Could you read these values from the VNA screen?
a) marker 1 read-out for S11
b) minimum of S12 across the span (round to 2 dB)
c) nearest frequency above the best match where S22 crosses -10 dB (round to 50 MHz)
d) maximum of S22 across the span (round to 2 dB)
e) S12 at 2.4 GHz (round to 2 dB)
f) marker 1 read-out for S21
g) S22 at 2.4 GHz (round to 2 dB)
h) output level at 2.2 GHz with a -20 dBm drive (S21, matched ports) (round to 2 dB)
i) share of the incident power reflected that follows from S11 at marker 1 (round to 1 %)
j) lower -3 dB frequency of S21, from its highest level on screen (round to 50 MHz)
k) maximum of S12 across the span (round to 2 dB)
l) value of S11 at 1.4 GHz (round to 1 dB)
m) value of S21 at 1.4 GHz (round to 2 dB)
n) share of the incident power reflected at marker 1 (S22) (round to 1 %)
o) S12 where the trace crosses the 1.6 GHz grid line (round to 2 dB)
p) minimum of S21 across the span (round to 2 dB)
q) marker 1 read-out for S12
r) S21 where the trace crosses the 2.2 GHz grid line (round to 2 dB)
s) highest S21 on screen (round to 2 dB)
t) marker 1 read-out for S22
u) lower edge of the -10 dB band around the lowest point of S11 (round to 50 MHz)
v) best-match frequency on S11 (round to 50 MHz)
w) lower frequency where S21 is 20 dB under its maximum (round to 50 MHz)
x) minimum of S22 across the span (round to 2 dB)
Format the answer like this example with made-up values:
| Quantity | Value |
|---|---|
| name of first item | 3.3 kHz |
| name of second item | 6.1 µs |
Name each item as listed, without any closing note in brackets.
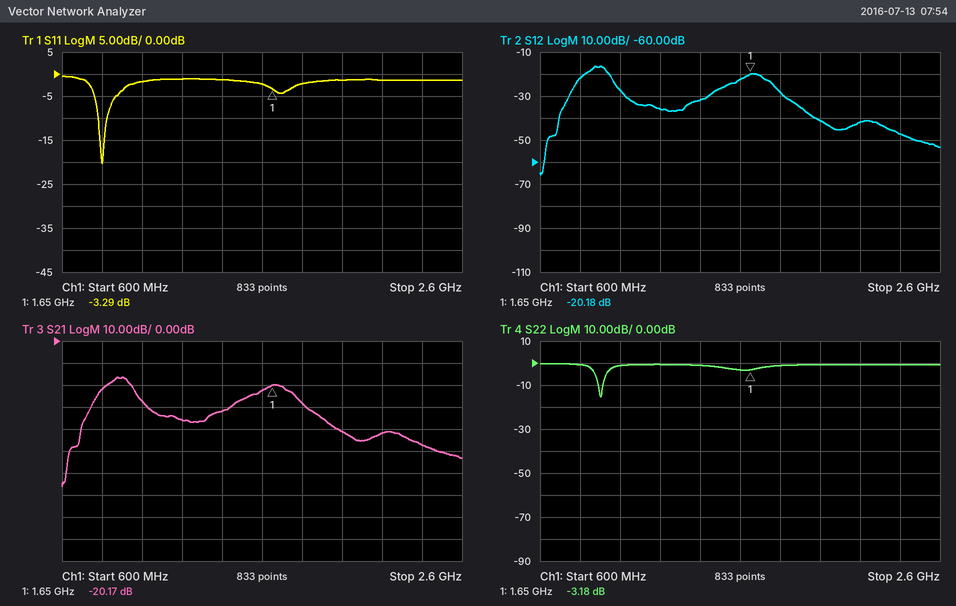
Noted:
| Quantity | Value |
|---|---|
| marker 1 read-out for S11 | -3.29 dB |
| minimum of S12 across the span | -66 dB |
| nearest frequency above the best match where S22 crosses -10 dB | 900 MHz |
| maximum of S22 across the span | 0 dB |
| S12 at 2.4 GHz | -48 dB |
| marker 1 read-out for S21 | -20.17 dB |
| S22 at 2.4 GHz | 0 dB |
| output level at 2.2 GHz with a -20 dBm drive (S21, matched ports) | -62 dBm |
| share of the incident power reflected that follows from S11 at marker 1 | 47 % |
| lower -3 dB frequency of S21, from its highest level on screen | 850 MHz |
| maximum of S12 across the span | -16 dB |
| value of S11 at 1.4 GHz | -1 dB |
| value of S21 at 1.4 GHz | -32 dB |
| share of the incident power reflected at marker 1 (S22) | 48 % |
| S12 where the trace crosses the 1.6 GHz grid line | -22 dB |
| minimum of S21 across the span | -66 dB |
| marker 1 read-out for S12 | -20.18 dB |
| S21 where the trace crosses the 2.2 GHz grid line | -42 dB |
| highest S21 on screen | -16 dB |
| marker 1 read-out for S22 | -3.18 dB |
| lower edge of the -10 dB band around the lowest point of S11 | 800 MHz |
| best-match frequency on S11 | 800 MHz |
| lower frequency where S21 is 20 dB under its maximum | 700 MHz |
| minimum of S22 across the span | -16 dB |
